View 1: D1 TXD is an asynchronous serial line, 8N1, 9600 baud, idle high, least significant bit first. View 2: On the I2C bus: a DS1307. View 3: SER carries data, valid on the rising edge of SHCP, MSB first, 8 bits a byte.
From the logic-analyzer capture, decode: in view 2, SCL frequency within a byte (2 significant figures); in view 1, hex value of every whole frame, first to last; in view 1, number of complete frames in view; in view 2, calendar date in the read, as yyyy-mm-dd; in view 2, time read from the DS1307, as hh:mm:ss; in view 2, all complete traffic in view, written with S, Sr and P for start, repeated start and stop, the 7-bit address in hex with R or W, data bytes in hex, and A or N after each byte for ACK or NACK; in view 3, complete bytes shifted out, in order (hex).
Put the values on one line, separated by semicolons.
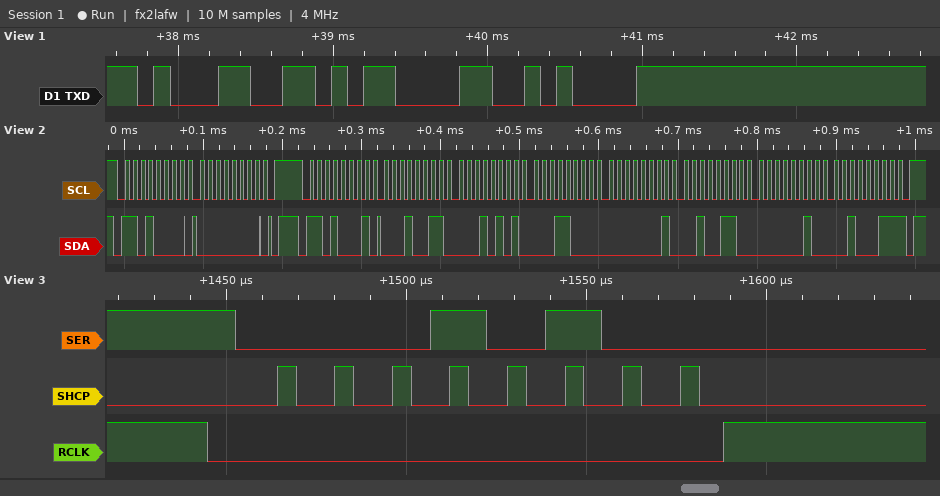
100 kHz; 31 0D 0A; 3; 2023-02-26; 18:15:13; S 68W A 00 A P S 68R A 13 A 15 A 18 A 01 A 26 A 02 A 23 N P; 0x14
